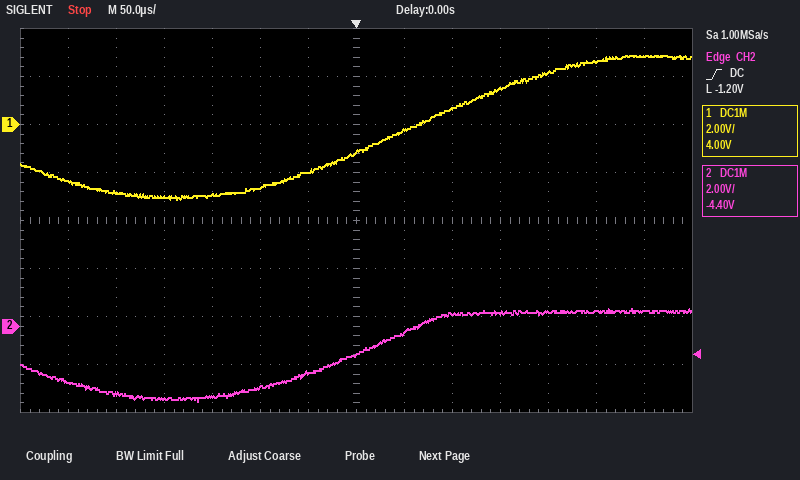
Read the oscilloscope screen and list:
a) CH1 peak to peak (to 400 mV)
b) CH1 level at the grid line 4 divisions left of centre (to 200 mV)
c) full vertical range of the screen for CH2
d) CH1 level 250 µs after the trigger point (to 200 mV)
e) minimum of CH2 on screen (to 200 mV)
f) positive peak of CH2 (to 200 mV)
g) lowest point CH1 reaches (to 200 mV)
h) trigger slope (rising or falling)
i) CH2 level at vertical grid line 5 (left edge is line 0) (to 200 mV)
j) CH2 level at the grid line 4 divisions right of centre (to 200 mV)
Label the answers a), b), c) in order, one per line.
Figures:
a) 6.0 V
b) -3.0 V
c) 16 V
d) 2.6 V
e) -3.2 V
f) 800 mV
g) -3.2 V
h) rising
i) -2.6 V
j) 600 mV
